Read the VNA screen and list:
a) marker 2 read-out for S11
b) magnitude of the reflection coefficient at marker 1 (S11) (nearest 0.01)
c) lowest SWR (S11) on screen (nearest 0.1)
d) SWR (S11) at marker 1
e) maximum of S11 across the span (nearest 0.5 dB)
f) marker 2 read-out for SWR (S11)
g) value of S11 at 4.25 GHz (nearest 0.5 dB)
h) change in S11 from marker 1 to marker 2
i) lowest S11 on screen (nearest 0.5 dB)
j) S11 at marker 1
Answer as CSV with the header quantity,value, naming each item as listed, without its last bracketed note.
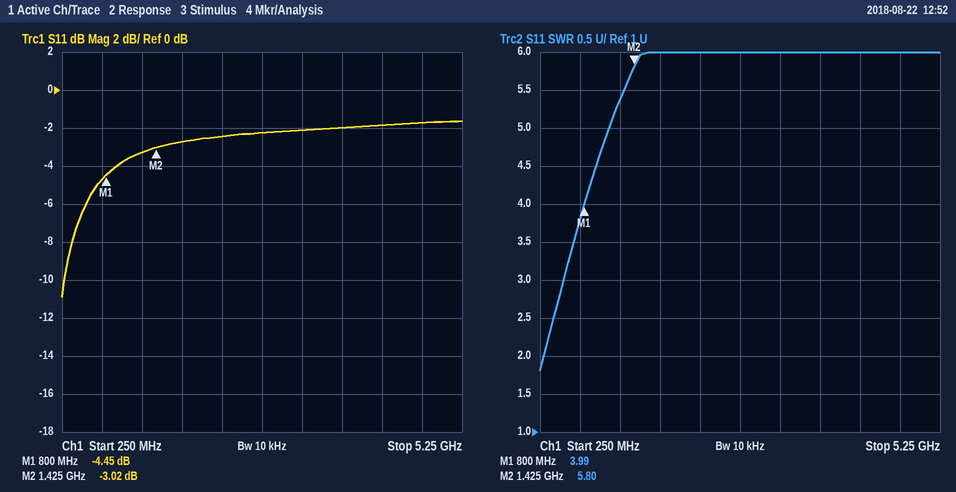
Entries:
quantity,value
marker 2 read-out for S11,-3.02 dB
magnitude of the reflection coefficient at marker 1 (S11),0.60
lowest SWR (S11) on screen,1.8
SWR (S11) at marker 1,3.99
maximum of S11 across the span,-1.5 dB
marker 2 read-out for SWR,5.80
value of S11 at 4.25 GHz,-2.0 dB
change in S11 from marker 1 to marker 2,1.43 dB
lowest S11 on screen,-11.0 dB
S11 at marker 1,-4.45 dB
